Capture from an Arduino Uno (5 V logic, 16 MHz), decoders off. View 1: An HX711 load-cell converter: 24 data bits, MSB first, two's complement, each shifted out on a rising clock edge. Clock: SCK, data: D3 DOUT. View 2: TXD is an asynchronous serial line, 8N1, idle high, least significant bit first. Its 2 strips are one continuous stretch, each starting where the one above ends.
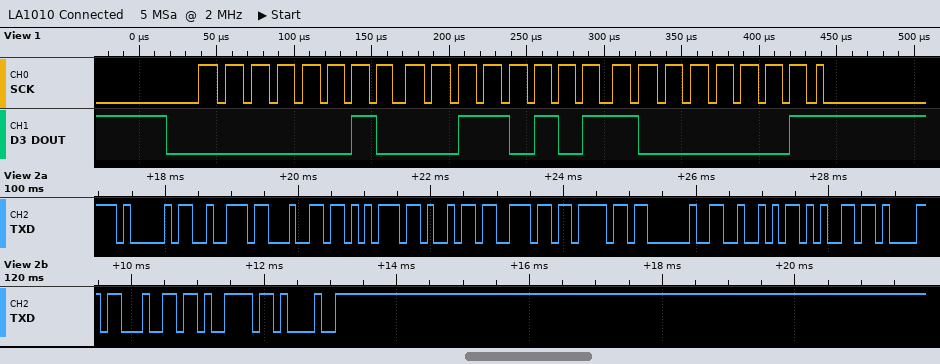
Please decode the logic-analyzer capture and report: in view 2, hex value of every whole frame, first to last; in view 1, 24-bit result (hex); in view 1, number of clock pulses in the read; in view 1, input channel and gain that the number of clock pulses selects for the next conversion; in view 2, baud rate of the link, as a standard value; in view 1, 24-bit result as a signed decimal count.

0x41 0x72 0x64 0x75 0x69 0x6E 0x6F 0x20 0x52 0x65 0x61 0x64 0x79 0x21
0x023581
25
channel A, gain 128
9600 baud
144769
